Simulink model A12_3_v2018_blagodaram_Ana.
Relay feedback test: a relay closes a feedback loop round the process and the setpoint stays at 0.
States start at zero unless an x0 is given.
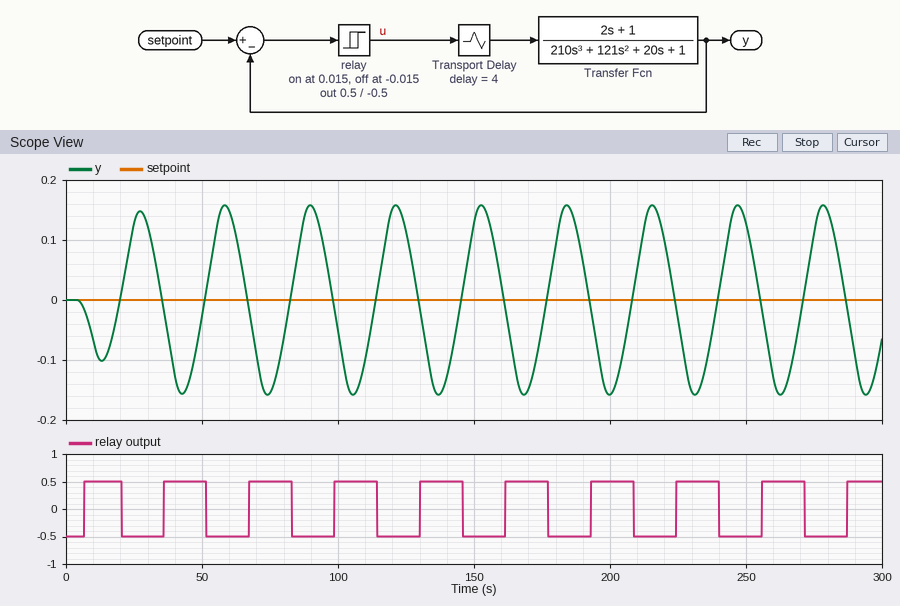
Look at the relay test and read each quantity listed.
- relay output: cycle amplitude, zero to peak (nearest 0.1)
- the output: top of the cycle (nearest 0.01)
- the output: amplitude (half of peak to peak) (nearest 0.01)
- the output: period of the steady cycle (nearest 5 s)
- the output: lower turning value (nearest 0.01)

0.5
0.16
0.16
30 s
-0.16
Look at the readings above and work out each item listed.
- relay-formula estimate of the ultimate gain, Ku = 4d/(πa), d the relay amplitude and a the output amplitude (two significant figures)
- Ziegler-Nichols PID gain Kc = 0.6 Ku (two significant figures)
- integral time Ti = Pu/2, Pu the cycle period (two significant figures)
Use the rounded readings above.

4.0
2.4
15 s
